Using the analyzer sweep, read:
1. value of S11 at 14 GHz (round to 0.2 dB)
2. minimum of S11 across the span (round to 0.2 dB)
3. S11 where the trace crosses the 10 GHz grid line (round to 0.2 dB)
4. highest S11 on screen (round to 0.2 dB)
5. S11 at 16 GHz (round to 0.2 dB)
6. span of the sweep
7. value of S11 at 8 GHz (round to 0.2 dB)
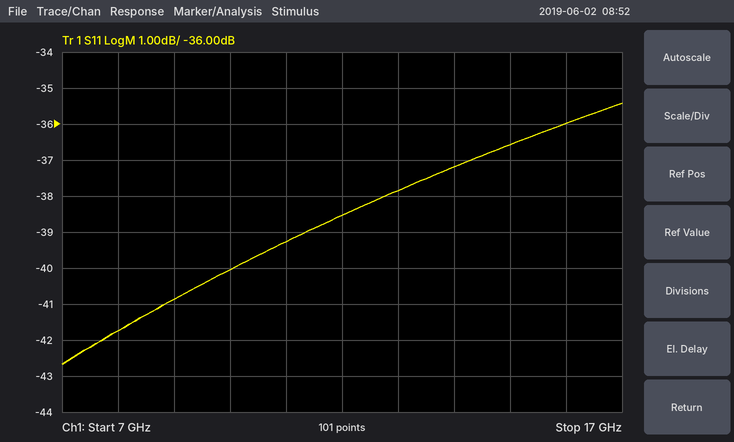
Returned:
-37.2 dB
-42.6 dB
-40.0 dB
-35.4 dB
-36.0 dB
10 GHz
-41.8 dB
